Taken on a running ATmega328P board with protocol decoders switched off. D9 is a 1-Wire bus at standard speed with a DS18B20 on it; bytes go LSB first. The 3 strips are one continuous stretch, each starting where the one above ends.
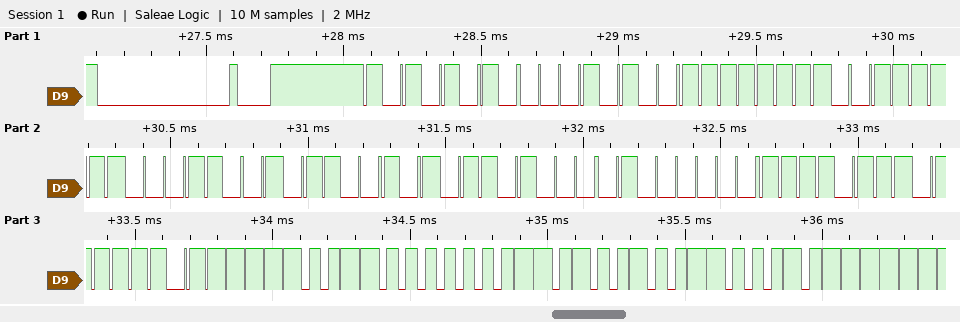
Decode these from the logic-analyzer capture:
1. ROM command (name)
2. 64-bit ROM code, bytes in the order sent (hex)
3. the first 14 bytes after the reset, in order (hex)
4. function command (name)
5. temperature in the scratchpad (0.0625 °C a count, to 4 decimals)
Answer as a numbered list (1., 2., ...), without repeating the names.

1. Match ROM
2. 28 FF FC 98 A6 16 02 EF
3. 55 28 FF FC 98 A6 16 02 EF BE 9F 01 4B 46
4. Read Scratchpad
5. 25.9375 °C
